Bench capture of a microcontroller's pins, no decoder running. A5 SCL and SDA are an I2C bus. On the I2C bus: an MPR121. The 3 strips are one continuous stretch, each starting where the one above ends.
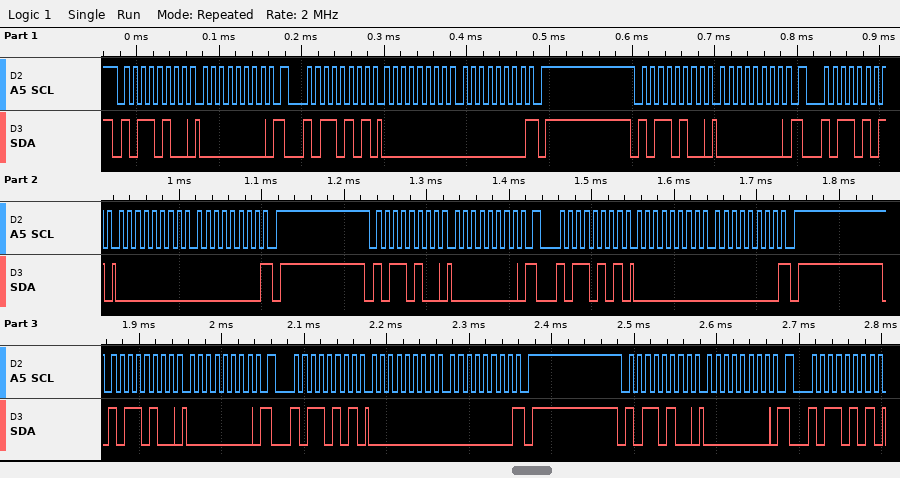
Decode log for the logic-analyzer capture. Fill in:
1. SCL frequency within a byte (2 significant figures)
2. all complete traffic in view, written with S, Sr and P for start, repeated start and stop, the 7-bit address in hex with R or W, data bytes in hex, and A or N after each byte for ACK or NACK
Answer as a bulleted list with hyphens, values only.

- 100 kHz
- S 5AW A 00 A Sr 5AR A 00 A 00 N P S 5AW A 00 A Sr 5AR A 00 A 00 N P S 5AW A 00 A Sr 5AR A 00 A 00 N P S 5AW A 00 A Sr 5AR A 00 A 00 N P S 5AW A 00 A Sr 5AR A
